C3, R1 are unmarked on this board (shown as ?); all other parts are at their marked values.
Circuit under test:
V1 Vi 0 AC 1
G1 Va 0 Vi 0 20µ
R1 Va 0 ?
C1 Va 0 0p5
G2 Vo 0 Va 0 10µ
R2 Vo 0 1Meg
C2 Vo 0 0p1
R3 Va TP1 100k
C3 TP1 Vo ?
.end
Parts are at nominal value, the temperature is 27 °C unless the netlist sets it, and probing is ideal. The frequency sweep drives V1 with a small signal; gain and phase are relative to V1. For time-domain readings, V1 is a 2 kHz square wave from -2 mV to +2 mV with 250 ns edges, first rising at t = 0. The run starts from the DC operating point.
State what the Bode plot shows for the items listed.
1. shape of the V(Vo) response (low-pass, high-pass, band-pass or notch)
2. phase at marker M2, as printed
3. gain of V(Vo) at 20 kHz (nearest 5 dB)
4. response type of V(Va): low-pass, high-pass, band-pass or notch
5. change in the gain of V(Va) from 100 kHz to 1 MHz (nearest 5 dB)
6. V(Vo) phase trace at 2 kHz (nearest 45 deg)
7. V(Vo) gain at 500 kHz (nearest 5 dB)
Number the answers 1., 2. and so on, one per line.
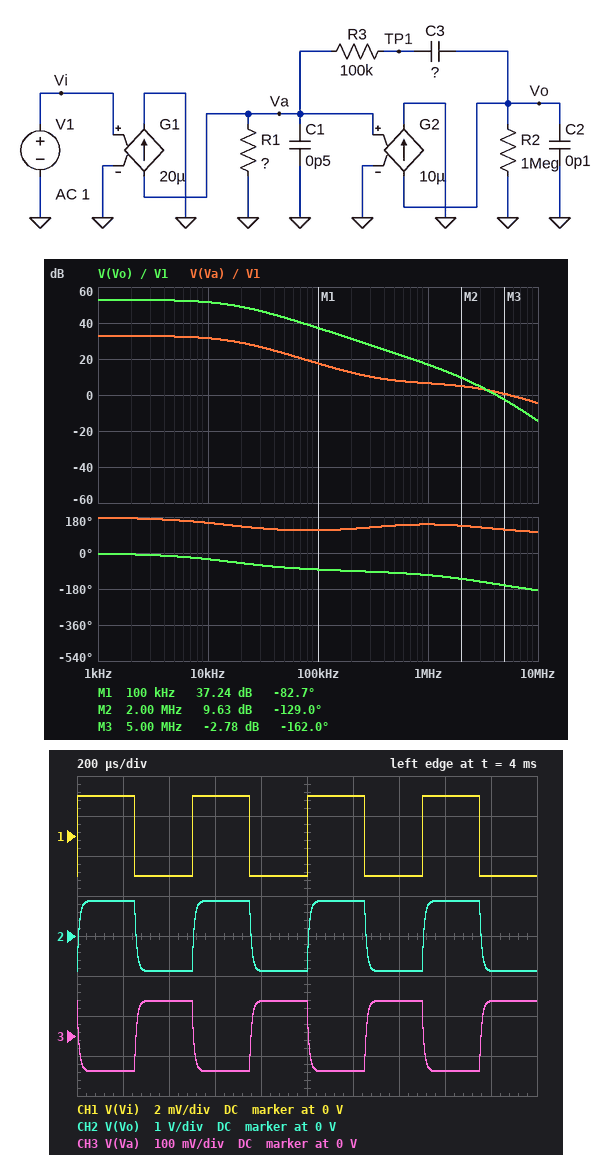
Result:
1. low-pass
2. -129.0 deg
3. 50 dB
4. low-pass
5. -10 dB
6. 0 deg
7. 25 dB
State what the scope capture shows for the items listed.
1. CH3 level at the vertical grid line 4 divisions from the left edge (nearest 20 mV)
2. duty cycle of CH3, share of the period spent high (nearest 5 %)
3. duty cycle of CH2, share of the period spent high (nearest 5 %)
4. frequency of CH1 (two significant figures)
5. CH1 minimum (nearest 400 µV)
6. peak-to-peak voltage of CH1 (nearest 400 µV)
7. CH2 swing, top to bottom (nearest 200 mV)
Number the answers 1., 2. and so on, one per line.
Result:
1. 80 mV
2. 50 %
3. 50 %
4. 2.0 kHz
5. -2.0 mV
6. 4.0 mV
7. 1.8 V
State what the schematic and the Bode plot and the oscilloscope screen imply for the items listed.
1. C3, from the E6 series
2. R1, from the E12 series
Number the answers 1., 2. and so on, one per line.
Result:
1. 330 fF
2. 2.2 MΩ
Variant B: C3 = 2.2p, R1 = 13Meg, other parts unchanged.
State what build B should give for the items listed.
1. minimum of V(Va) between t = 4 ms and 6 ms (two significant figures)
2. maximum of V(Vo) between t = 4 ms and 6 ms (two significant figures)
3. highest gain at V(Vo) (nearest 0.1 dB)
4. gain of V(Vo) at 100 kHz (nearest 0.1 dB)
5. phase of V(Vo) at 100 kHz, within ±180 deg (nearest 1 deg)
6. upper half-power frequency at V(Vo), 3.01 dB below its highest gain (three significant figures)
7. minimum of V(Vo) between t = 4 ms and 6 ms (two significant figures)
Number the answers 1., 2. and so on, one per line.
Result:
1. -190 mV
2. 1.9 V
3. 68.3 dB
4. 22.1 dB
5. -92 deg
6. 492 Hz
7. -1.9 V
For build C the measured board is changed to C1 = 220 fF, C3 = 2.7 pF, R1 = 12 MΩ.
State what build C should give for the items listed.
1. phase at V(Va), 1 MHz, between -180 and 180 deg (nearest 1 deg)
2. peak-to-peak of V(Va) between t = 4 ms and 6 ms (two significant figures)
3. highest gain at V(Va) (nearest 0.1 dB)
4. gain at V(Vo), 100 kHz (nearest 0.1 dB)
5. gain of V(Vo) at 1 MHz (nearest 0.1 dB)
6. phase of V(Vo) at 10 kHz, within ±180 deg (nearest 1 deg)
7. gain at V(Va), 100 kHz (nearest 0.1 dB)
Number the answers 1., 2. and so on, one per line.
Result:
1. 169 deg
2. 320 mV
3. 47.6 dB
4. 20.5 dB
5. 0.4 dB
6. -88 deg
7. 7.2 dB
